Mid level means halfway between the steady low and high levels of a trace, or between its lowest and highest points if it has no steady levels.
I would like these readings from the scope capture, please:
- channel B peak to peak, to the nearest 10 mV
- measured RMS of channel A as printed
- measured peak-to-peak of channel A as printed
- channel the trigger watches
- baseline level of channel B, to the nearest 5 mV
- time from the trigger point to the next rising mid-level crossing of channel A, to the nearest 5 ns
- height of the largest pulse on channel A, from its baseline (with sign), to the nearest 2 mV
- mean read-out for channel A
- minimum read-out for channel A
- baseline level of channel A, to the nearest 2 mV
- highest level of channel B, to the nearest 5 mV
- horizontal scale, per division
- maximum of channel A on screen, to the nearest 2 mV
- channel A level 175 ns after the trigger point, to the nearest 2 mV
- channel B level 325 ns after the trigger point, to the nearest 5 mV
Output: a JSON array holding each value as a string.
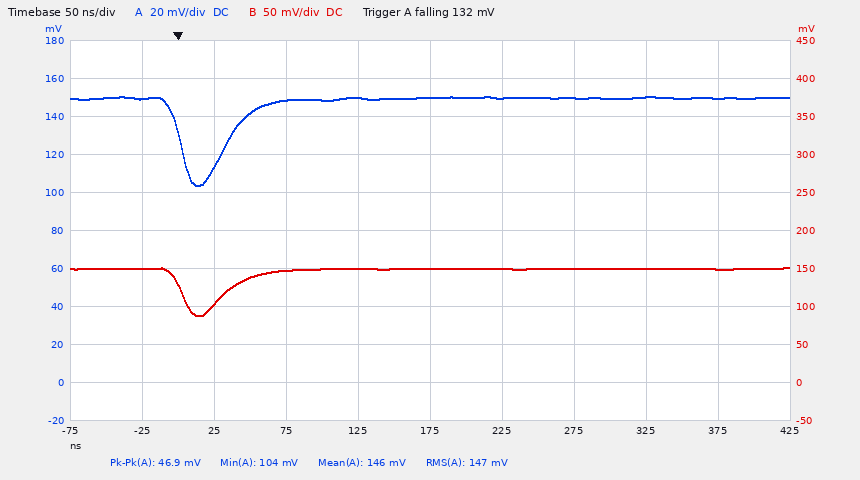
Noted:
["60 mV", "147 mV", "46.9 mV", "channel A", "150 mV", "35 ns", "-46 mV", "146 mV", "104 mV", "150 mV", "150 mV", "50 ns", "150 mV", "150 mV", "150 mV"]
